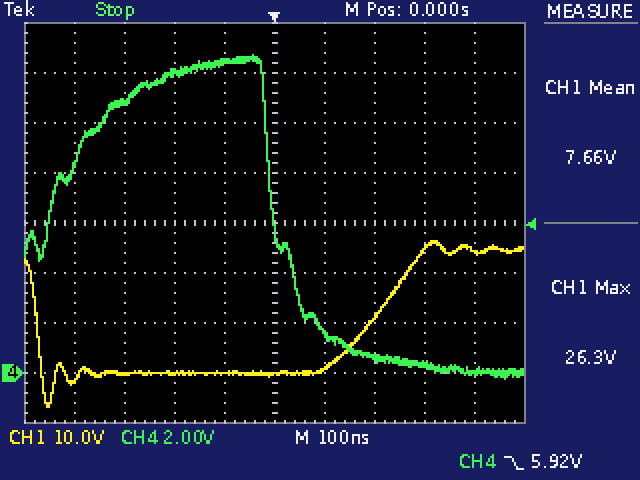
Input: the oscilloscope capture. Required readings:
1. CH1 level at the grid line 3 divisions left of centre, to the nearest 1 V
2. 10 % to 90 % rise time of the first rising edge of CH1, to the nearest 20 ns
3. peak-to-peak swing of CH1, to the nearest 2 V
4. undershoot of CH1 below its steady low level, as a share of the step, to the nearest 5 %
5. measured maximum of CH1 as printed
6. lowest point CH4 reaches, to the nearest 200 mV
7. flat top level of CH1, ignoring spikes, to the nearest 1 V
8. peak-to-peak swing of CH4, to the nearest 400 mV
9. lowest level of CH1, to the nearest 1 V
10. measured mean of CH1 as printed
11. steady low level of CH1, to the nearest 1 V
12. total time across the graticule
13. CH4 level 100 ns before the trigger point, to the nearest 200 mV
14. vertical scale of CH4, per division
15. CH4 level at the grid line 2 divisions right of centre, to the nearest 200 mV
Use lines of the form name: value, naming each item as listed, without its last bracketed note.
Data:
CH1 level at the grid line 3 divisions left of centre, to the nearest 1 V: 0 V
10 % to 90 % rise time of the first rising edge of CH1, to the nearest 20 ns: 160 ns
peak-to-peak swing of CH1, to the nearest 2 V: 34 V
undershoot of CH1 below its steady low level, as a share of the step, to the nearest 5 %: 30 %
measured maximum of CH1 as printed: 26.3 V
lowest point CH4 reaches, to the nearest 200 mV: -200 mV
flat top level of CH1, ignoring spikes, to the nearest 1 V: 25 V
peak-to-peak swing of CH4, to the nearest 400 mV: 12.8 V
lowest level of CH1, to the nearest 1 V: -7 V
measured mean of CH1 as printed: 7.66 V
steady low level of CH1, to the nearest 1 V: 0 V
total time across the graticule: 1 µs
CH4 level 100 ns before the trigger point, to the nearest 200 mV: 12.4 V
vertical scale of CH4, per division: 2 V
CH4 level at the grid line 2 divisions right of centre, to the nearest 200 mV: 600 mV
